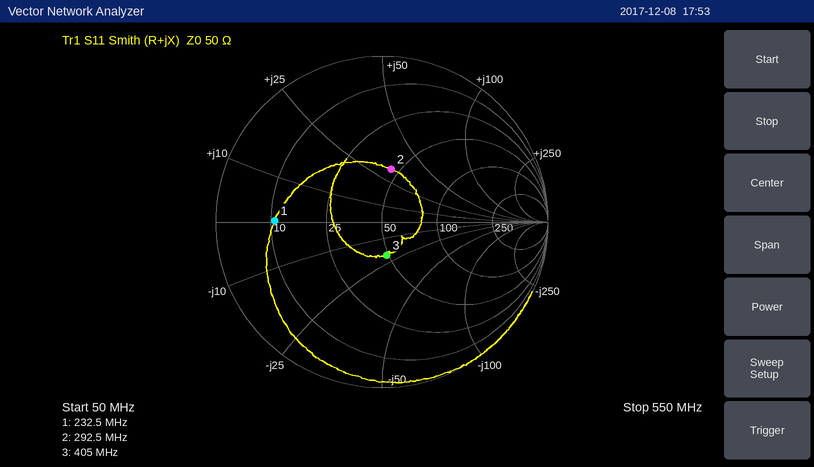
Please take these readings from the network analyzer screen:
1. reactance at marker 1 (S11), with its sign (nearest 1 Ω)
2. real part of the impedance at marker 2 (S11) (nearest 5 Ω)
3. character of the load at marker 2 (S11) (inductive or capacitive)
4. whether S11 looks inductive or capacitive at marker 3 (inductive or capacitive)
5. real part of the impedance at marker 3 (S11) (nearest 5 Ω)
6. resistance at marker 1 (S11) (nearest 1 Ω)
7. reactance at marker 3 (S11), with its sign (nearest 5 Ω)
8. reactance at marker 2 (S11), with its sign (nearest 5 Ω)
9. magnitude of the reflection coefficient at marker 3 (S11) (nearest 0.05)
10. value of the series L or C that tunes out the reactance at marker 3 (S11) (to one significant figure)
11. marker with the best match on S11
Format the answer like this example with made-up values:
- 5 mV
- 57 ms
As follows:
- 0 Ω
- 45 Ω
- inductive
- capacitive
- 50 Ω
- 11 Ω
- -20 Ω
- +30 Ω
- 0.20
- 8 nH
- marker 3
